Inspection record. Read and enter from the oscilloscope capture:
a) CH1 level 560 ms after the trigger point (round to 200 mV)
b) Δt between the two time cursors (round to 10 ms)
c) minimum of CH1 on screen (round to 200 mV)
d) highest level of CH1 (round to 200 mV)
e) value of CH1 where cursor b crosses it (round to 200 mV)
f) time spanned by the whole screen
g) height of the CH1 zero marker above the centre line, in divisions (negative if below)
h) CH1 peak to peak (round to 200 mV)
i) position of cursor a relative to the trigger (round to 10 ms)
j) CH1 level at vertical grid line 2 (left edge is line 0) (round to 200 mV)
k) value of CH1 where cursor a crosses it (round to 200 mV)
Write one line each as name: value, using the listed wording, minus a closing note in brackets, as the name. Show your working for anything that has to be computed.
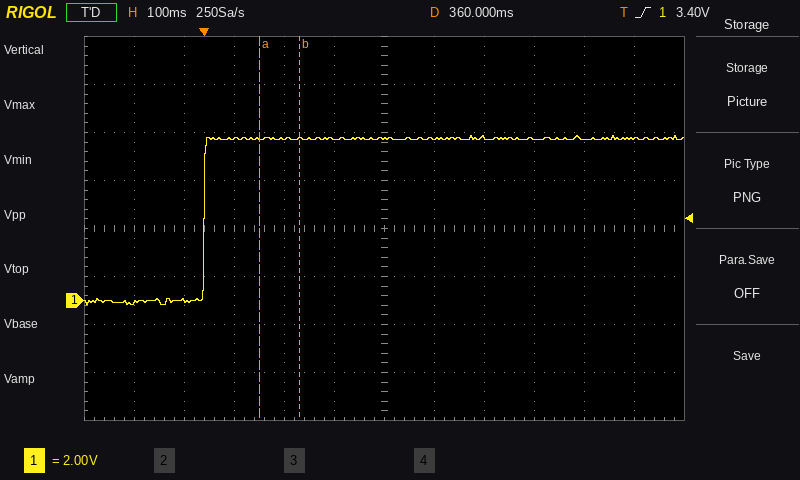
CH1 level 560 ms after the trigger point: 6.8 V
Δt between the two time cursors: 80 ms
minimum of CH1 on screen: -200 mV
highest level of CH1: 6.8 V
value of CH1 where cursor b crosses it: 6.8 V
time spanned by the whole screen: 1.2 s
height of the CH1 zero marker above the centre line, in divisions: -1.5 div
CH1 peak to peak: 6.8 V − (-200 mV) = 7.0 V
position of cursor a relative to the trigger: +110 ms
CH1 level at vertical grid line 2 (left edge is line 0): 0.0 V
value of CH1 where cursor a crosses it: 6.8 V
